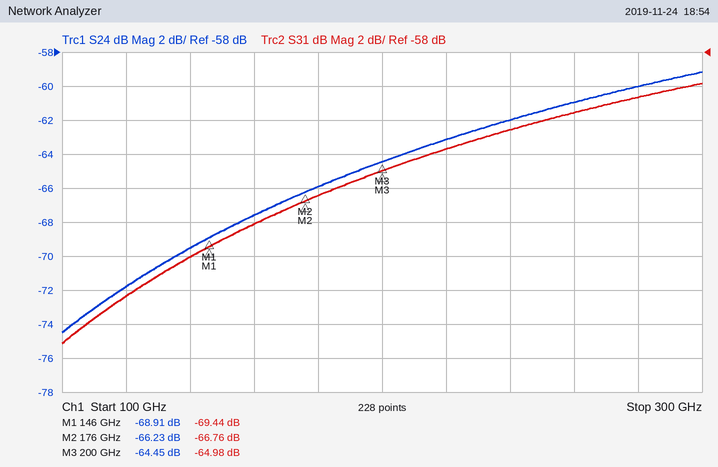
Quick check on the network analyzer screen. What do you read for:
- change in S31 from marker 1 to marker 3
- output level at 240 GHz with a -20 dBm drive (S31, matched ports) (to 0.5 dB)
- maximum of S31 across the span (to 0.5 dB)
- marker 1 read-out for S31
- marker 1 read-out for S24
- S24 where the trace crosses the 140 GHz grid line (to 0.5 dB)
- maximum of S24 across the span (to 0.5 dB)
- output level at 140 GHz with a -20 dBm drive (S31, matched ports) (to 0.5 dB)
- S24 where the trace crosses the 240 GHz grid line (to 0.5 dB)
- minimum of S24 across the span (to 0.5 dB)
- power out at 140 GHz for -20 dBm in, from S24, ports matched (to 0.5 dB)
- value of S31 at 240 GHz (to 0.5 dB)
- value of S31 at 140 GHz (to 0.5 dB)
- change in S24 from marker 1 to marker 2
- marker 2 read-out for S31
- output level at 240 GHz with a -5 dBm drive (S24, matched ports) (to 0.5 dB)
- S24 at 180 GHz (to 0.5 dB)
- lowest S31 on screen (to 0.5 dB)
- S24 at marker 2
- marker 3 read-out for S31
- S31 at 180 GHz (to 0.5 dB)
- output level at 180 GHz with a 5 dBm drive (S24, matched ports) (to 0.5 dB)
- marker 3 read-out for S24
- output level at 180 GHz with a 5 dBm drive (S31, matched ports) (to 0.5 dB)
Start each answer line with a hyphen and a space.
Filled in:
- 4.46 dB
- -82.5 dBm
- -60.0 dB
- -69.44 dB
- -68.91 dB
- -69.5 dB
- -59.0 dB
- -90.0 dBm
- -62.0 dB
- -74.5 dB
- -89.5 dBm
- -62.5 dB
- -70.0 dB
- 2.68 dB
- -66.76 dB
- -67.0 dBm
- -66.0 dB
- -75.0 dB
- -66.23 dB
- -64.98 dB
- -66.5 dB
- -61.0 dBm
- -64.45 dB
- -61.5 dBm
